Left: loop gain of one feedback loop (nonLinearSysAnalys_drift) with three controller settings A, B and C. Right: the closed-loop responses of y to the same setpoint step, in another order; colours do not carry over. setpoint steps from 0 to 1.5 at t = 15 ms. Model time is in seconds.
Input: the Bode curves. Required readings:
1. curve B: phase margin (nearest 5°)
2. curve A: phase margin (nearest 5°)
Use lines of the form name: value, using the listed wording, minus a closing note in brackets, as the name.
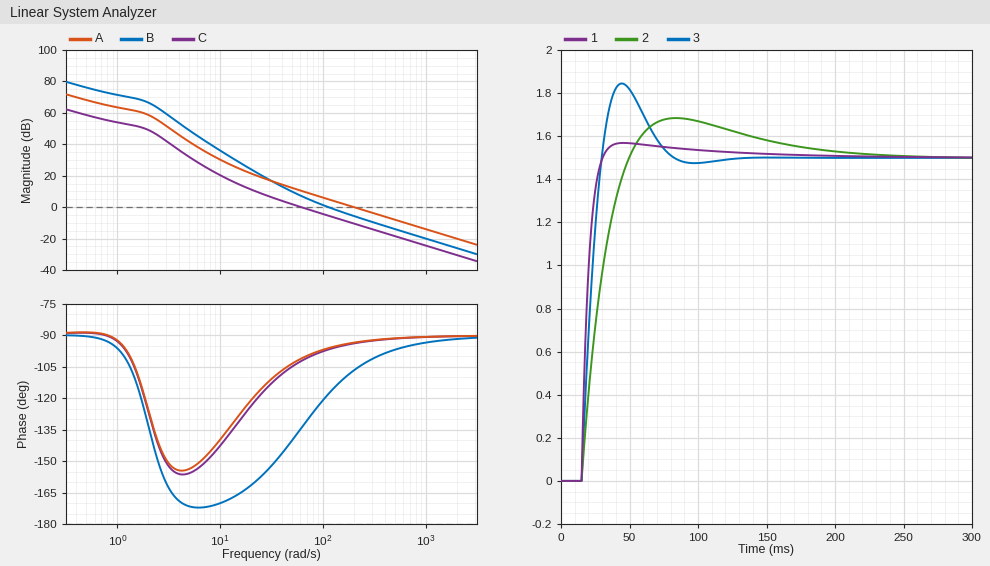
curve B: phase margin: 60°
curve A: phase margin: 85°
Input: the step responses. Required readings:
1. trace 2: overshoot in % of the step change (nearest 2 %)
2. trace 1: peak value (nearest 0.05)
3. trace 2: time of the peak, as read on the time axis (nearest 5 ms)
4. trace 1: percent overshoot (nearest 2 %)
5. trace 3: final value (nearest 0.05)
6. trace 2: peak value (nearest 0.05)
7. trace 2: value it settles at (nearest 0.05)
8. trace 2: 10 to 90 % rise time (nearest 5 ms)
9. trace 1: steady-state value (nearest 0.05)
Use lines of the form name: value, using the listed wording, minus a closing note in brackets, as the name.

trace 2: overshoot in % of the step change: 12 %
trace 1: peak value: 1.55
trace 2: time of the peak, as read on the time axis: 85 ms
trace 1: percent overshoot: 4 %
trace 3: final value: 1.50
trace 2: peak value: 1.70
trace 2: value it settles at: 1.50
trace 2: 10 to 90 % rise time: 25 ms
trace 1: steady-state value: 1.50
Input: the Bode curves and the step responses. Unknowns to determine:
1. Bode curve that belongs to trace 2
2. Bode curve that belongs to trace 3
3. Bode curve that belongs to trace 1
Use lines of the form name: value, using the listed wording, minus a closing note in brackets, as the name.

Bode curve that belongs to trace 2: C
Bode curve that belongs to trace 3: B
Bode curve that belongs to trace 1: A
